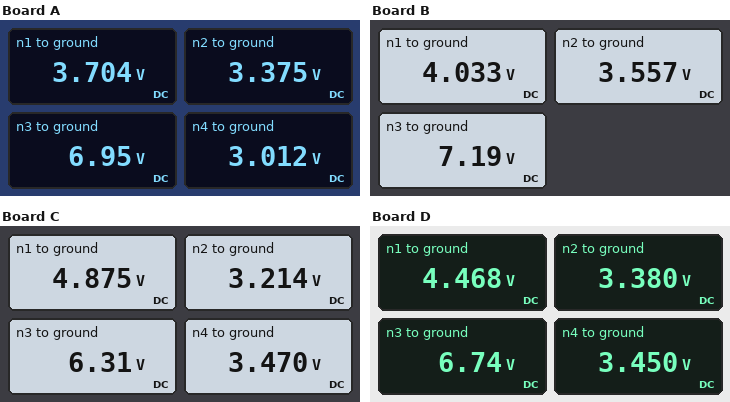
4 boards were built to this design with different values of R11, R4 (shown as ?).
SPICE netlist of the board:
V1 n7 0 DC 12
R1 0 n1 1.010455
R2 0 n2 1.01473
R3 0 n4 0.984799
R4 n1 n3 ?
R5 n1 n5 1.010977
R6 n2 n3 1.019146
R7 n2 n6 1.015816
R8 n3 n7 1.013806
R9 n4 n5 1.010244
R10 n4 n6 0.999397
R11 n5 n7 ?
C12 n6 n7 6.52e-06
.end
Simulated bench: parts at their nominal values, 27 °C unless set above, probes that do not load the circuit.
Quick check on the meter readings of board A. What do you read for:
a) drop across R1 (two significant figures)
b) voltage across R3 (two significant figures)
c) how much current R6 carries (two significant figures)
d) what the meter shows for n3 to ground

3.7 V
3.0 V
3.5 A
6.95 V
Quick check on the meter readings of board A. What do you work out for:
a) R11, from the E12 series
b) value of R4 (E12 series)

1.2 Ω
2.2 Ω
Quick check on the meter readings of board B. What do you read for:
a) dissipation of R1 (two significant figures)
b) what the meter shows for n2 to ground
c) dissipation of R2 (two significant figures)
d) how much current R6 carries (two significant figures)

16 W
3.557 V
12 W
3.6 A
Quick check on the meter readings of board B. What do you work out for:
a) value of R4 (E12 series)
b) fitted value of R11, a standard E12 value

2.7 Ω
0.82 Ω
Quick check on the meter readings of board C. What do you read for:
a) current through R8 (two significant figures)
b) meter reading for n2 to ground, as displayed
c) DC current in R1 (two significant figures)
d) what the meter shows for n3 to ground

5.6 A
3.214 V
4.8 A
6.31 V
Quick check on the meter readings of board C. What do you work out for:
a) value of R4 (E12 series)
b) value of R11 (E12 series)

0.56 Ω
0.82 Ω
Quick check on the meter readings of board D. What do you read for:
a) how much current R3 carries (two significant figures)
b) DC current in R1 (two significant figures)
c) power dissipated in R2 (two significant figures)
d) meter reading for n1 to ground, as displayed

3.5 A
4.4 A
11 W
4.468 V
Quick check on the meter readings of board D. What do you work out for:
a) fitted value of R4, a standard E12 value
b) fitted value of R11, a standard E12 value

1.2 Ω
0.82 Ω
